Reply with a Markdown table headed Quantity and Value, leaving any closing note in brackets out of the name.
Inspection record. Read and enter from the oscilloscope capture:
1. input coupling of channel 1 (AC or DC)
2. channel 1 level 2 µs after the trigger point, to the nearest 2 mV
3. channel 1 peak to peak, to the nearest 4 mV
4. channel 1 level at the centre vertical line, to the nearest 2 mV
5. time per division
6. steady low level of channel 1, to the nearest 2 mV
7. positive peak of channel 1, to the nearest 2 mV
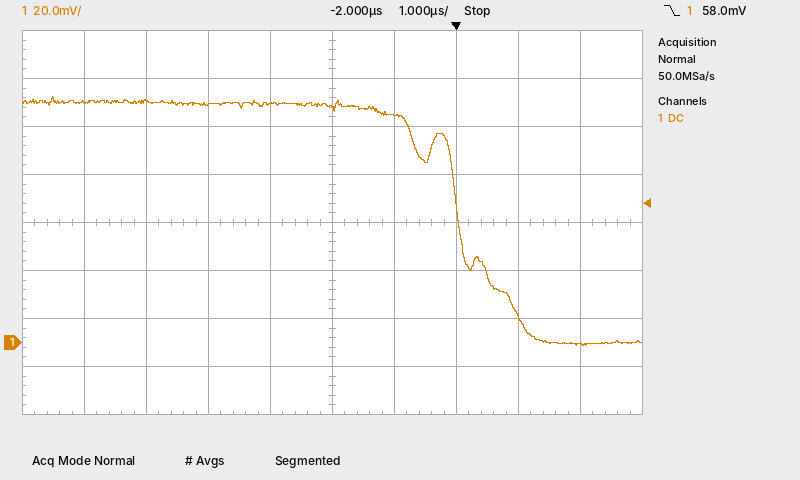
| Quantity | Value |
|---|---|
| input coupling of channel 1 | DC |
| channel 1 level 2 µs after the trigger point, to the nearest 2 mV | 0 mV |
| channel 1 peak to peak, to the nearest 4 mV | 104 mV |
| channel 1 level at the centre vertical line, to the nearest 2 mV | 98 mV |
| time per division | 1 µs |
| steady low level of channel 1, to the nearest 2 mV | 0 mV |
| positive peak of channel 1, to the nearest 2 mV | 102 mV |
